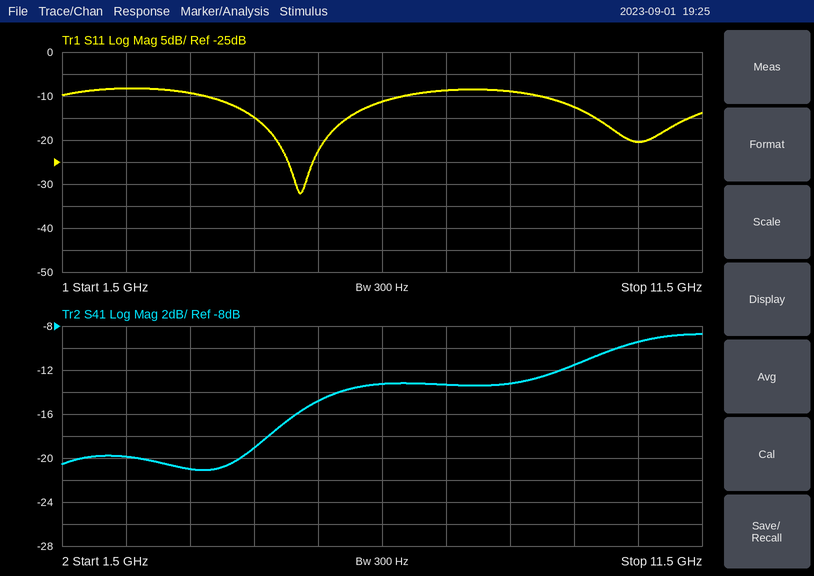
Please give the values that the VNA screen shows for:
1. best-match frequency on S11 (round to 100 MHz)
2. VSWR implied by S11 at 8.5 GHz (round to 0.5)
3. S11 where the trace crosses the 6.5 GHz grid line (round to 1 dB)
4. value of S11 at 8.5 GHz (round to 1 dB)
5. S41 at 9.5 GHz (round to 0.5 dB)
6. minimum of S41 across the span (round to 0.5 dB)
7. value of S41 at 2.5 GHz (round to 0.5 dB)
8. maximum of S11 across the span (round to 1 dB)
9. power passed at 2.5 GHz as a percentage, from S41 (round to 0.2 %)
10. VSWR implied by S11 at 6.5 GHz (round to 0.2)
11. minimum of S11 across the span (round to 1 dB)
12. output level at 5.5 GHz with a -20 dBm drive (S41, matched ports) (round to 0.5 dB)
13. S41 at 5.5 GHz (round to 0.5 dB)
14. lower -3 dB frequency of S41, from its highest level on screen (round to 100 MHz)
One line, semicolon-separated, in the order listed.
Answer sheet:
5.2 GHz; 2.0; -11 dB; -9 dB; -11.5 dB; -21.0 dB; -20.0 dB; -8 dB; 1.0 %; 1.8; -32 dB; -35.0 dBm; -15.0 dB; 9.4 GHz
